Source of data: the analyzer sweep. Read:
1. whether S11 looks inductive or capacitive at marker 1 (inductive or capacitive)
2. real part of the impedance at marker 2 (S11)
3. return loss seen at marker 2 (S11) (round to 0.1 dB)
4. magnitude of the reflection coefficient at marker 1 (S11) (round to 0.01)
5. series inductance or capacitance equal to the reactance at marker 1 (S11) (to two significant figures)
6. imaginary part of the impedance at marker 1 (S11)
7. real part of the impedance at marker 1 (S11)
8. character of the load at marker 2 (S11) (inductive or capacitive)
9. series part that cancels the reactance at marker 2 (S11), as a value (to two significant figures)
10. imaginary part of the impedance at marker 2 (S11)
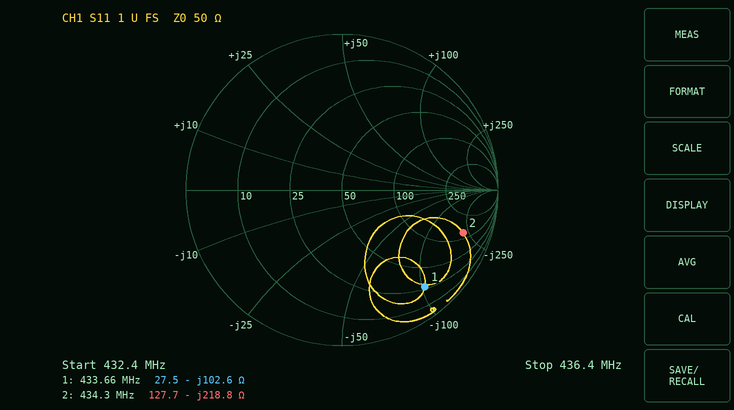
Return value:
capacitive
127.7 Ω
1.7 dB
0.82
3.6 pF
-102.6 Ω
27.5 Ω
capacitive
80 nH
-218.8 Ω
